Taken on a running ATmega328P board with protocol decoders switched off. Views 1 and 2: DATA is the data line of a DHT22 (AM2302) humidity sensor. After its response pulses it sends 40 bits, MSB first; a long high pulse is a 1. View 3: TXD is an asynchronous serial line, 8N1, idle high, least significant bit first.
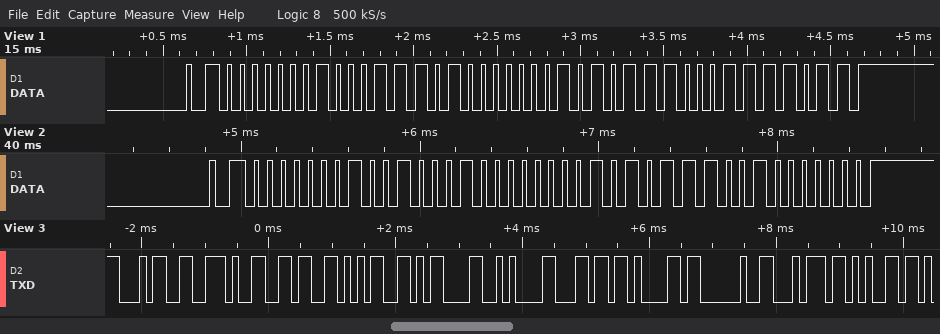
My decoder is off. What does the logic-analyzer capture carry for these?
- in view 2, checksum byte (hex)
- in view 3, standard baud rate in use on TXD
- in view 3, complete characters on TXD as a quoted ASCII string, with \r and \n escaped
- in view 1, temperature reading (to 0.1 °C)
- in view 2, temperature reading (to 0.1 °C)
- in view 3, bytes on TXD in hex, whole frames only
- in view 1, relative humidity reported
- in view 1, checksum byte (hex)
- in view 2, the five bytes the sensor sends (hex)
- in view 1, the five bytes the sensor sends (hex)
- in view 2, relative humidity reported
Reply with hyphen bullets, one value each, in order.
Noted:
- 0x80
- 9600 baud
- "4.65\r\nla te"
- 34.8 °C
- 34.8 °C
- 34 2E 36 35 0D 0A 6C 61 20 74 65
- 28.5 %
- 0x7B
- 01 22 01 5C 80
- 01 1D 01 5C 7B
- 29.0 %
